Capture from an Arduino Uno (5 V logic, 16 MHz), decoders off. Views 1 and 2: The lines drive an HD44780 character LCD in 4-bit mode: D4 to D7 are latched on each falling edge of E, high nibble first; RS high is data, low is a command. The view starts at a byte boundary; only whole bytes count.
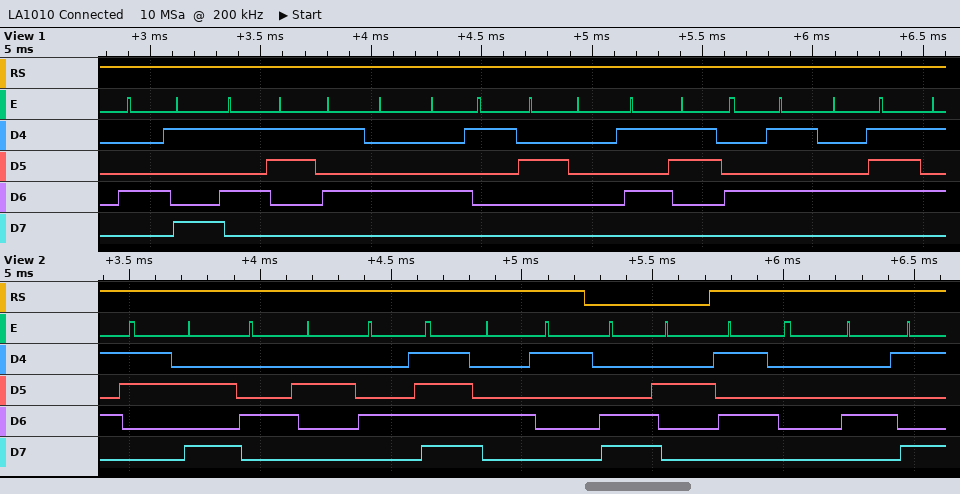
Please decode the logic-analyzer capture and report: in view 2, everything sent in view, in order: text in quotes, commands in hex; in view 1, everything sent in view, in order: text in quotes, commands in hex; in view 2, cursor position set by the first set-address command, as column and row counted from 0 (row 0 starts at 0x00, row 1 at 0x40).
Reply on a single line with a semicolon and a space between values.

":BOA" 0xC2 "PI"; "ISTA SEG"; column 2, row 1
